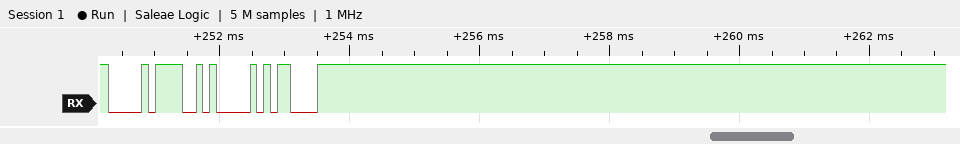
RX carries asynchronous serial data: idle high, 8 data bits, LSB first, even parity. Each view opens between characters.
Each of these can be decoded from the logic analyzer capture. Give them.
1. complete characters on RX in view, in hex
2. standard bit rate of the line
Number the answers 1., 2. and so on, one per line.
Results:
1. D0, 0A, 0D
2. 9600 baud
